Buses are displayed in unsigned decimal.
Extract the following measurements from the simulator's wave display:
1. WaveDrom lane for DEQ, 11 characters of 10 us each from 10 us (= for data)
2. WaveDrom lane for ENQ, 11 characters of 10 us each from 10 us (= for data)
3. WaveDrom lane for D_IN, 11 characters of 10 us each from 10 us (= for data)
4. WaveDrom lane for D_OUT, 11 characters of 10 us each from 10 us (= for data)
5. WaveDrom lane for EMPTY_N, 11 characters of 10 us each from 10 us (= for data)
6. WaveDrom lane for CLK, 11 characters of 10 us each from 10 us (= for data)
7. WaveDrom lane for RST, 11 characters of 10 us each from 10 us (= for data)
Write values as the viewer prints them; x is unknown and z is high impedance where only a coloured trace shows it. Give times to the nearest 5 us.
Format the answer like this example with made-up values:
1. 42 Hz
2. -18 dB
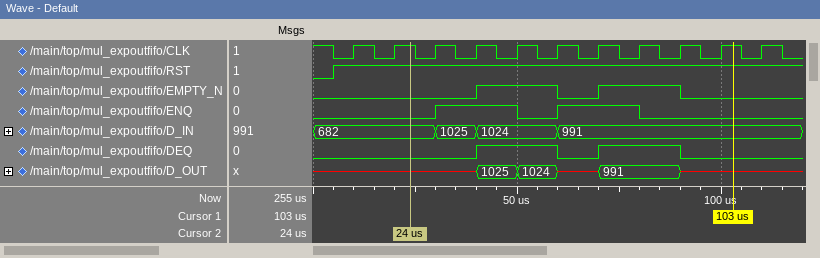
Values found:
1. {name: 'DEQ', wave: '0..1.01.0..'}
2. {name: 'ENQ', wave: '0.1.01.0...'}
3. {name: 'D_IN', wave: '=.==.=.....', data: '682 1025 1024 991'}
4. {name: 'D_OUT', wave: 'x..==x=.x..', data: '1025 1024 991'}
5. {name: 'EMPTY_N', wave: '0..1.01.0..'}
6. {name: 'CLK', wave: 'p..........'}
7. {name: 'RST', wave: '1..........'}
